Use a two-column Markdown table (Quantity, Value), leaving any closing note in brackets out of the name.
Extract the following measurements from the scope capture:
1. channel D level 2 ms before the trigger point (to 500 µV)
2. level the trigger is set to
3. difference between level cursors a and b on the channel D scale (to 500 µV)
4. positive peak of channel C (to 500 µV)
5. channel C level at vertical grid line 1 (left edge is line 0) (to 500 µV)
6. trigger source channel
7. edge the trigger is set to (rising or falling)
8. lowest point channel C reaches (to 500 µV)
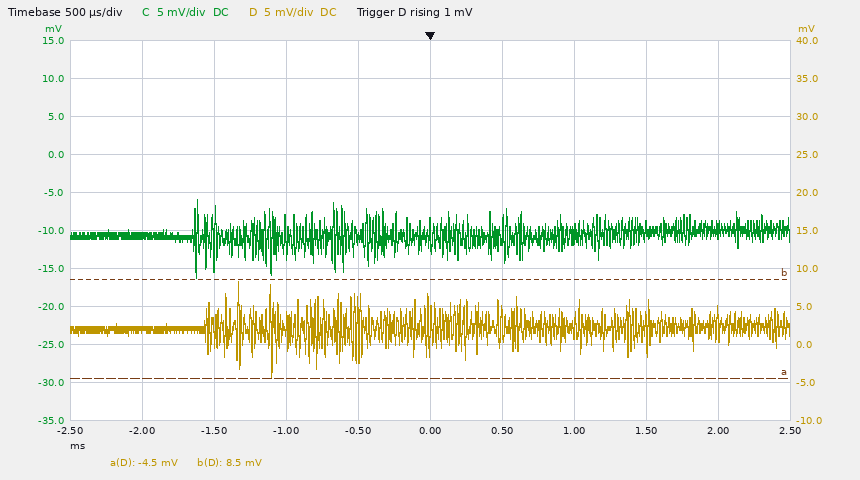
| Quantity | Value |
|---|---|
| channel D level 2 ms before the trigger point | 2.0 mV |
| level the trigger is set to | 1 mV |
| difference between level cursors a and b on the channel D scale | 13.0 mV |
| positive peak of channel C | -6.0 mV |
| channel C level at vertical grid line 1 (left edge is line 0) | -10.5 mV |
| trigger source channel | channel D |
| edge the trigger is set to | rising |
| lowest point channel C reaches | -16.0 mV |
